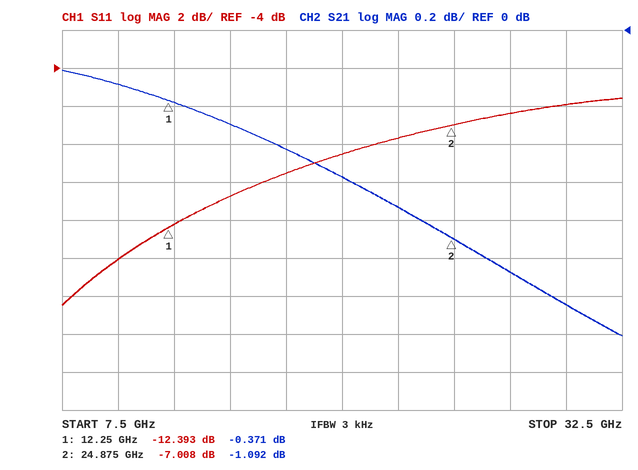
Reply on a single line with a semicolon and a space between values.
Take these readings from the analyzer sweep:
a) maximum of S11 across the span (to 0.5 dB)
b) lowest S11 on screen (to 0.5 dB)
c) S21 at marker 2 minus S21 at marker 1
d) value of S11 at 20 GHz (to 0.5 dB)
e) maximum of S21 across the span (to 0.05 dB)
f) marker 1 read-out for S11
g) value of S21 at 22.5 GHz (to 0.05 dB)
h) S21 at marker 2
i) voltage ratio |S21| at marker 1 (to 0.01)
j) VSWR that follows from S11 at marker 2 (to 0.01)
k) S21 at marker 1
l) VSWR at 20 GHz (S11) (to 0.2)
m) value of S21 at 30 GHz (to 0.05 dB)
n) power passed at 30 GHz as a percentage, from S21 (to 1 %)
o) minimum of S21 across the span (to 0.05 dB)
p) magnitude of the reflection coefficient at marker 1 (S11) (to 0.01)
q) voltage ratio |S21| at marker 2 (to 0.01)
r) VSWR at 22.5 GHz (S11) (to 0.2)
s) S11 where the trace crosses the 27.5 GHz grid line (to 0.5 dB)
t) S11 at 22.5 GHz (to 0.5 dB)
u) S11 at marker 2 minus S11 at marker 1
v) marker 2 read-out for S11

-5.5 dB; -16.5 dB; -0.721 dB; -8.5 dB; -0.20 dB; -12.393 dB; -0.95 dB; -1.092 dB; 0.96; 2.61; -0.371 dB; 2.2; -1.45 dB; 72 %; -1.60 dB; 0.24; 0.88; 2.4; -6.5 dB; -7.5 dB; 5.385 dB; -7.008 dB
